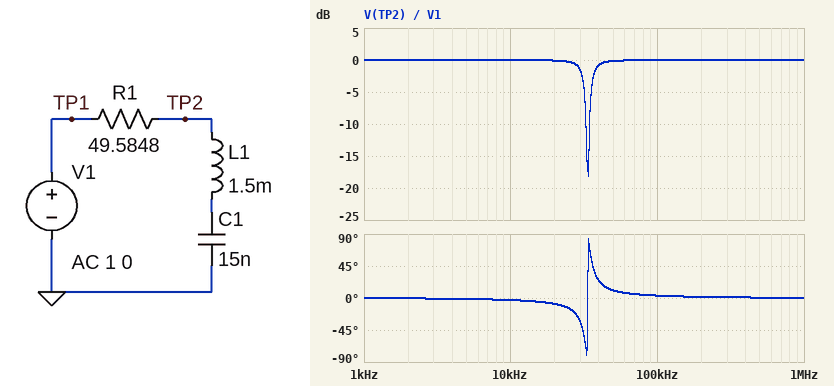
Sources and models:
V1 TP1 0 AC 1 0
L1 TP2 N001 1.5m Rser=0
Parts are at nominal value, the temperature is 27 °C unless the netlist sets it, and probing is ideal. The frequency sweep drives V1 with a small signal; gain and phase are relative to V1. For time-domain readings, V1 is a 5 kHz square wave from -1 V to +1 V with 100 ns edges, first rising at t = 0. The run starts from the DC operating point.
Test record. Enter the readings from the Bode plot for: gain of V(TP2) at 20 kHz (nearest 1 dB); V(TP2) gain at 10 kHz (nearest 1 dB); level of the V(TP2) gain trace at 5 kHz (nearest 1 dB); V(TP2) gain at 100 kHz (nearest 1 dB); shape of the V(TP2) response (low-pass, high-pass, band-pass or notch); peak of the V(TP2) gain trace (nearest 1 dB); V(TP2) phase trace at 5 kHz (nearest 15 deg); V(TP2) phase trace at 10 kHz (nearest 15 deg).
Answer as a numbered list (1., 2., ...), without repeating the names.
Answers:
1. 0 dB
2. 0 dB
3. 0 dB
4. 0 dB
5. notch
6. 0 dB
7. 0 deg
8. 0 deg
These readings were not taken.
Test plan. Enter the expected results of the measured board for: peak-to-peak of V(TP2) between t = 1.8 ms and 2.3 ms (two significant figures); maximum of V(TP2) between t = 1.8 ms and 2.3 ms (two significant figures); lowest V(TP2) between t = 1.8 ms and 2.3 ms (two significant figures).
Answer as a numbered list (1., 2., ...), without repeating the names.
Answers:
1. 2.5 V
2. 1.2 V
3. -1.2 V
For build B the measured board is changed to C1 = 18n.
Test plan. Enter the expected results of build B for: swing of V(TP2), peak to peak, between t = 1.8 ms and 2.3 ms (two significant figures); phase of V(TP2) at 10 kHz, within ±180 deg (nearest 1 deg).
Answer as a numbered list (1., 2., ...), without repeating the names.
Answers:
1. 2.4 V
2. -4 deg
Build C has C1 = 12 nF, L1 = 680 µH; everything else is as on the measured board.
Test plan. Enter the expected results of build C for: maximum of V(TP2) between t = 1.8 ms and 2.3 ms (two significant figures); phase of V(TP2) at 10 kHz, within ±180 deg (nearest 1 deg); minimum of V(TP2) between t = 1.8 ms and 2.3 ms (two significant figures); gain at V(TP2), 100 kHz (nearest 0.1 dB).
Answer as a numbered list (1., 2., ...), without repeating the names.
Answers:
1. 1.3 V
2. -2 deg
3. -1.3 V
4. -0.1 dB
